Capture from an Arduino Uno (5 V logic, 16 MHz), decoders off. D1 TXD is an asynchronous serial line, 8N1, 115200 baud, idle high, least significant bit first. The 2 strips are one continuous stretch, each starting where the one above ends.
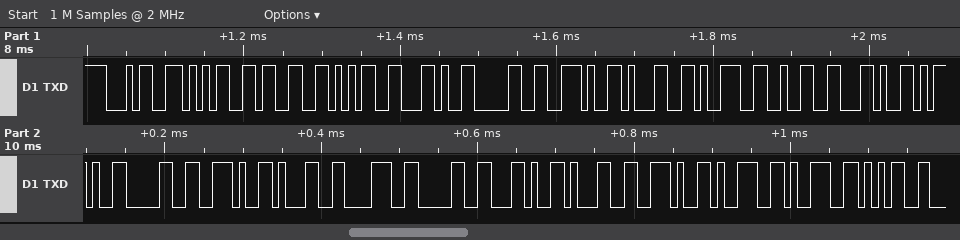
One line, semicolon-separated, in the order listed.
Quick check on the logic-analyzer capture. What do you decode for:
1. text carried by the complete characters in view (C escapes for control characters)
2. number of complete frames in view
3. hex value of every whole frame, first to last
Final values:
"4535,0.192,-0.180,1.995"; 23; 34 35 33 35 2C 30 2E 31 39 32 2C 2D 30 2E 31 38 30 2C 31 2E 39 39 35
